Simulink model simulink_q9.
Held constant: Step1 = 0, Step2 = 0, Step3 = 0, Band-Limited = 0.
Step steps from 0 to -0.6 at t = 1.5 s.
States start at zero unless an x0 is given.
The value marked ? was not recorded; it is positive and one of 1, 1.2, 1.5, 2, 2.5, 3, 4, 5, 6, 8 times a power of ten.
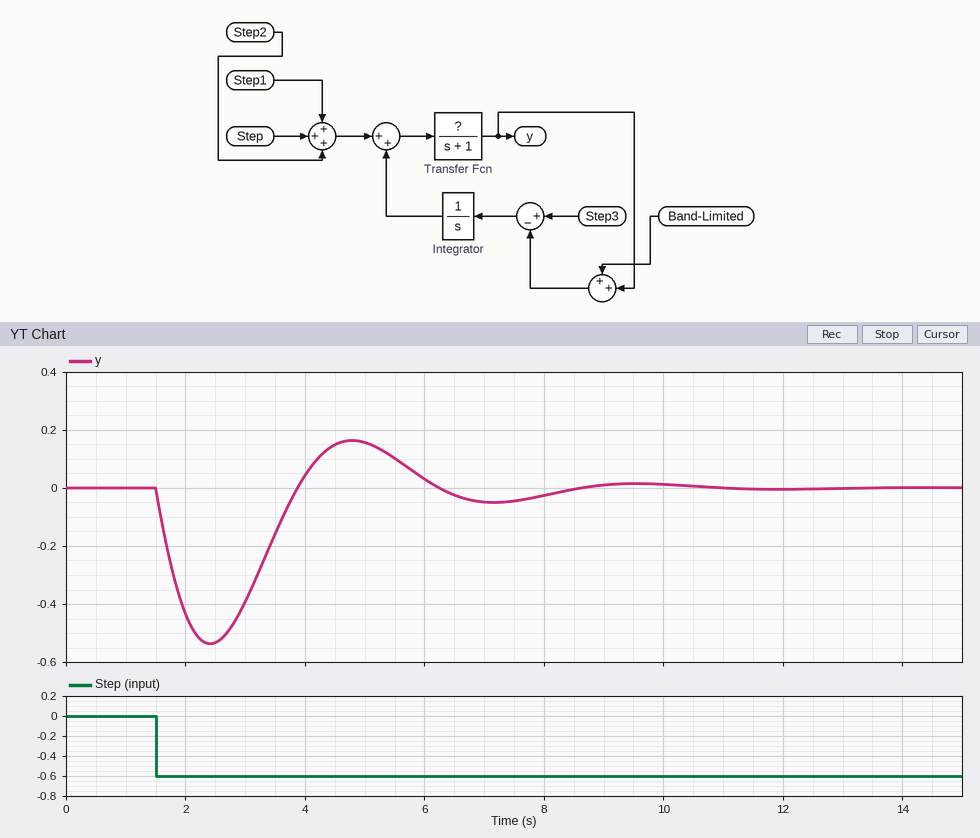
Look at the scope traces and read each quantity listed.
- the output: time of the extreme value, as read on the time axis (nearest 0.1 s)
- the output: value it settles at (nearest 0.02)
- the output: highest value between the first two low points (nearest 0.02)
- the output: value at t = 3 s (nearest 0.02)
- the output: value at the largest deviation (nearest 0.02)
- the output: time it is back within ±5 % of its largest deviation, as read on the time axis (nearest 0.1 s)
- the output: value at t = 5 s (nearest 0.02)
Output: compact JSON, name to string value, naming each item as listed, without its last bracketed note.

{"the output: time of the extreme value, as read on the time axis": "2.4 s", "the output: value it settles at": "0.00", "the output: highest value between the first two low points": "0.16", "the output: value at t = 3 s": "-0.40", "the output: value at the largest deviation": "-0.54", "the output: time it is back within ±5 % of its largest deviation, as read on the time axis": "8.0 s", "the output: value at t = 5 s": "0.16"}
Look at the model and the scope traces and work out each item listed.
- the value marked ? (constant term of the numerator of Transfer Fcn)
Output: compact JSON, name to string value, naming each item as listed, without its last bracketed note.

{"the value marked ?": "2"}
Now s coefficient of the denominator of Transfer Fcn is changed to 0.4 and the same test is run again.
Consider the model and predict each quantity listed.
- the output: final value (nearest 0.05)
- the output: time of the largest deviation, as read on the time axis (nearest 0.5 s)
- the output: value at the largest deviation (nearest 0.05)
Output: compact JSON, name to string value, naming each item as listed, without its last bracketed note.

{"the output: final value": "0.00", "the output: time of the largest deviation, as read on the time axis": "2.0 s", "the output: value at the largest deviation": "-0.70"}
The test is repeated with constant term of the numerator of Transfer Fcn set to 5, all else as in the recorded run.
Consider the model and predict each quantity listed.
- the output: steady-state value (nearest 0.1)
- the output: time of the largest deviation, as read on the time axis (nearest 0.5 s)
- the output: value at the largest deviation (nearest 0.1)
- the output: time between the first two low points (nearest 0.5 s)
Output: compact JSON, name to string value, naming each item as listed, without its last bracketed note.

{"the output: steady-state value": "0.0", "the output: time of the largest deviation, as read on the time axis": "2.0 s", "the output: value at the largest deviation": "-1.0", "the output: time between the first two low points": "3.0 s"}
